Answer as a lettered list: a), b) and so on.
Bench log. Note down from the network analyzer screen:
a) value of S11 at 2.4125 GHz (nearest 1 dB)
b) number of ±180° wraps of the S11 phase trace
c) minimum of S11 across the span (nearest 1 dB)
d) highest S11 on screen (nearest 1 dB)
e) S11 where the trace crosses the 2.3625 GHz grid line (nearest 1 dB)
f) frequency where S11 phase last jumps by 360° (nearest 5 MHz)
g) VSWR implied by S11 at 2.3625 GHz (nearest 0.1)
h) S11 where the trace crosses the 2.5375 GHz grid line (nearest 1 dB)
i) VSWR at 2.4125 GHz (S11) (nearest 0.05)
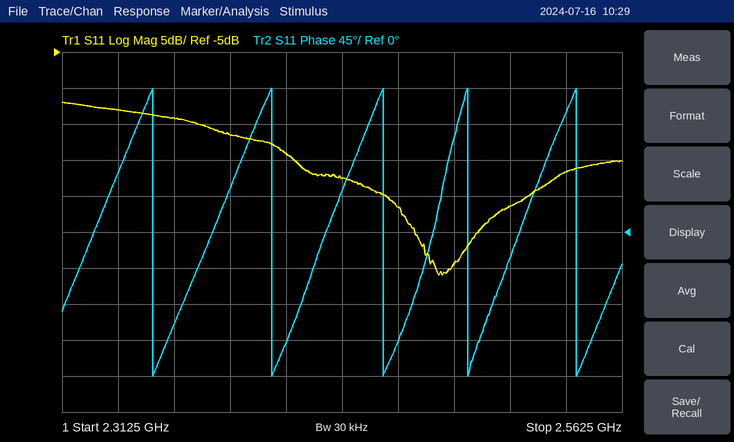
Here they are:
a) -19 dB
b) 5
c) -36 dB
d) -12 dB
e) -14 dB
f) 2.540 GHz
g) 1.5
h) -22 dB
i) 1.25
